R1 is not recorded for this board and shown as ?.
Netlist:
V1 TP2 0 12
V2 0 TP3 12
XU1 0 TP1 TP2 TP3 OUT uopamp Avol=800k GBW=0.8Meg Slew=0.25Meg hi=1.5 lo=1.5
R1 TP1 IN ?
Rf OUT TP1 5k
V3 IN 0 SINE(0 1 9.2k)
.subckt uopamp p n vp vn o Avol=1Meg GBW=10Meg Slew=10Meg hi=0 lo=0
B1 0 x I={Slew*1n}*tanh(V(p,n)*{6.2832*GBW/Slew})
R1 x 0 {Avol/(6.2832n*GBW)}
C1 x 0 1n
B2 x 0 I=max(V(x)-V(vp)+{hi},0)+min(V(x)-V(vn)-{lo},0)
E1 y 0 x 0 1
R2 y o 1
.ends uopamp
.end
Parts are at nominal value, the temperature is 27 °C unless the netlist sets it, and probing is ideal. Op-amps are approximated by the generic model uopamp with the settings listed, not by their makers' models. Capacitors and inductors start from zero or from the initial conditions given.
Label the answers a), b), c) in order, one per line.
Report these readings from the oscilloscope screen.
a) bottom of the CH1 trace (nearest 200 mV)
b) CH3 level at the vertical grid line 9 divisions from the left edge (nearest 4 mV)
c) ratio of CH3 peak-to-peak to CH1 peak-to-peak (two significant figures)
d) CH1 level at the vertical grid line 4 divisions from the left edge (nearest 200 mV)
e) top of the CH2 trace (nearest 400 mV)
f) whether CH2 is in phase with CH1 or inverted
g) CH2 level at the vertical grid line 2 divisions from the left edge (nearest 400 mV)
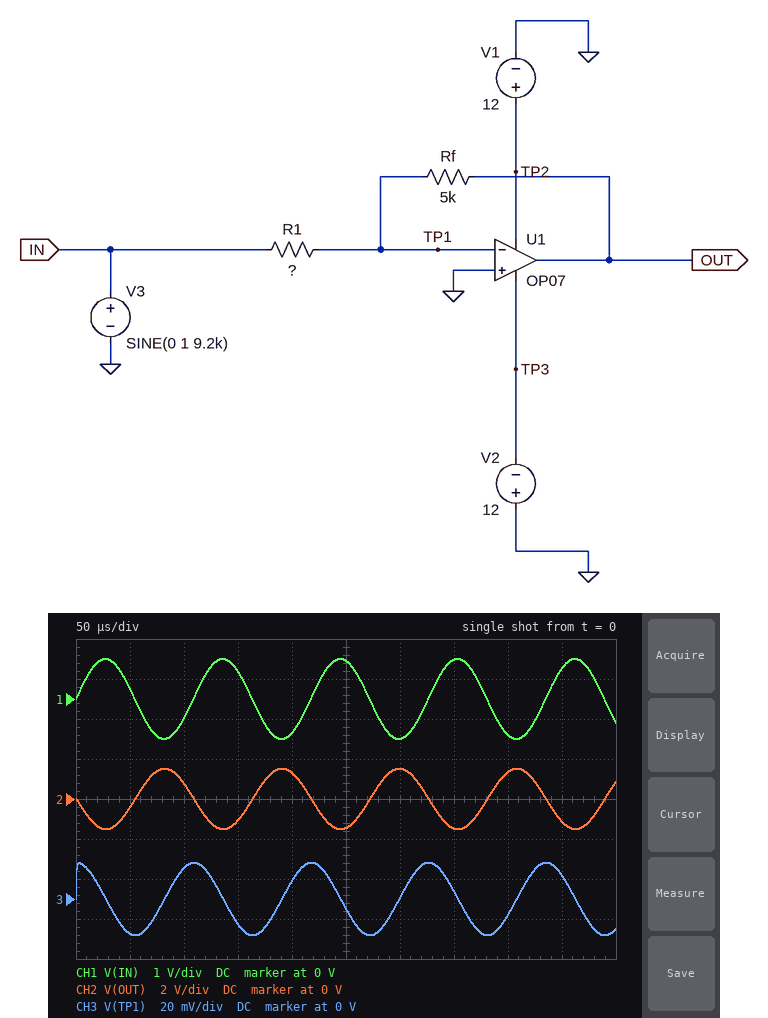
a) -1.0 V
b) 12 mV
c) 0.018
d) -800 mV
e) 1.6 V
f) inverted
g) 800 mV
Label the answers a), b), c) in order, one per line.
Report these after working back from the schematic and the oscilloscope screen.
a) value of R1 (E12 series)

a) 3.3 kΩ
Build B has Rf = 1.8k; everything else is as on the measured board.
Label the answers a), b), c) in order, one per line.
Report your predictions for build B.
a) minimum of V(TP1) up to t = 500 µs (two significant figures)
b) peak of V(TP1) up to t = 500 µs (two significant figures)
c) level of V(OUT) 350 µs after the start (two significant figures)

a) -6.3 mV
b) 6.3 mV
c) -530 mV
